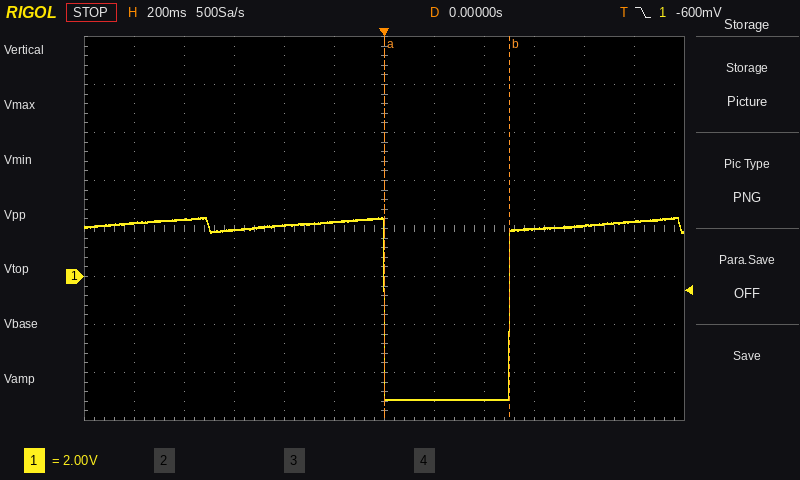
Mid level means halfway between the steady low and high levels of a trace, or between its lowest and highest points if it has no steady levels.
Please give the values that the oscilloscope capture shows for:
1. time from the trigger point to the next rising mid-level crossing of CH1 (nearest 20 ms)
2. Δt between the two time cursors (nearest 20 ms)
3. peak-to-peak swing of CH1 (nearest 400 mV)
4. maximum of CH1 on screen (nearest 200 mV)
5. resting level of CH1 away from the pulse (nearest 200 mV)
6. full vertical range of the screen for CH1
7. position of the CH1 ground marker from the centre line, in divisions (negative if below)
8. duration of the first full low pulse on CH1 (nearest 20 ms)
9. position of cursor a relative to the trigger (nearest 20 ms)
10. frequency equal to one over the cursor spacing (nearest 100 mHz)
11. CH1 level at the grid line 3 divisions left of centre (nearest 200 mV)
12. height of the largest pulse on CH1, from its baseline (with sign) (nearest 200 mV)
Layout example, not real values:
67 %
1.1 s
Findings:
500 ms
500 ms
7.6 V
2.4 V
2.2 V
16 V
-1.0 div
500 ms
0 ms
2.0 Hz
2.0 V
-7.2 V
